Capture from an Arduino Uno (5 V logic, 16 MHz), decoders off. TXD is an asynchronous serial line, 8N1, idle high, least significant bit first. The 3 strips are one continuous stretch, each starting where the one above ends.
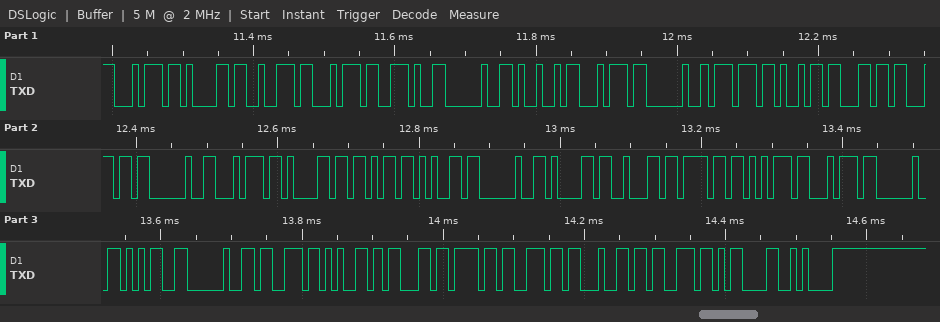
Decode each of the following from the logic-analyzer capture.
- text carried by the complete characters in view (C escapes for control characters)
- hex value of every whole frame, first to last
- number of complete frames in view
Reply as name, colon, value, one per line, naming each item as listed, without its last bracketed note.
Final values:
text carried by the complete characters in view: "tart. It will take about 5 seconds\r\n"
hex value of every whole frame, first to last: 0x74 0x61 0x72 0x74 0x2E 0x20 0x49 0x74 0x20 0x77 0x69 0x6C 0x6C 0x20 0x74 0x61 0x6B 0x65 0x20 0x61 0x62 0x6F 0x75 0x74 0x20 0x35 0x20 0x73 0x65 0x63 0x6F 0x6E 0x64 0x73 0x0D 0x0A
number of complete frames in view: 36
